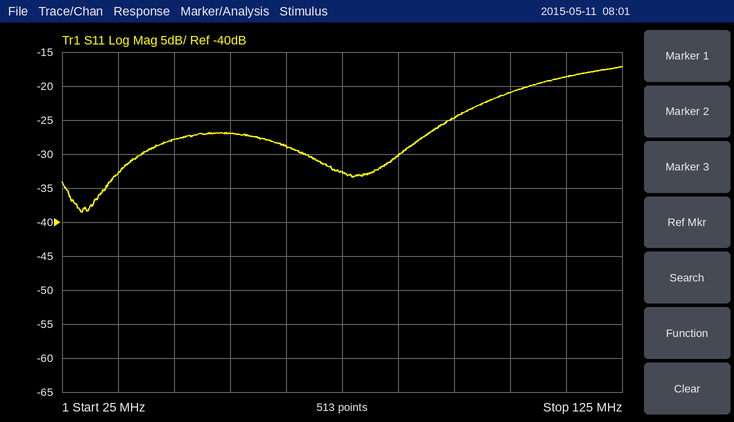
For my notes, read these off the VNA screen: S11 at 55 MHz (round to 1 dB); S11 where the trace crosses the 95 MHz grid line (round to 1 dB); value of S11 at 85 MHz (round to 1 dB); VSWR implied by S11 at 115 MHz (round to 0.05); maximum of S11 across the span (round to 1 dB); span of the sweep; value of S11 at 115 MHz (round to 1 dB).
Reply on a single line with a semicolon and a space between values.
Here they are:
-27 dB; -25 dB; -30 dB; 1.25; -17 dB; 100 MHz; -19 dB
